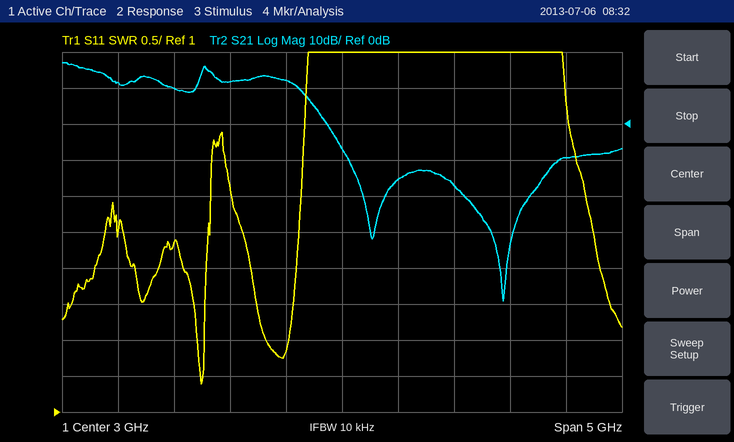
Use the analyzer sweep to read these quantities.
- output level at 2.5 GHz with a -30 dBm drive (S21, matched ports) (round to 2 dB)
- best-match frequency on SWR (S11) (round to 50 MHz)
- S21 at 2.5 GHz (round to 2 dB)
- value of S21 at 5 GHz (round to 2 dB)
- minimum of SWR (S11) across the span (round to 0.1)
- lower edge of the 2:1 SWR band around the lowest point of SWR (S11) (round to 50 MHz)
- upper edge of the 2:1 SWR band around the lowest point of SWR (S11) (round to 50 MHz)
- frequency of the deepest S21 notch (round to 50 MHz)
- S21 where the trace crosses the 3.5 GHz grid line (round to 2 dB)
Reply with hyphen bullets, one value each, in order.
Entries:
- -18 dBm
- 1.75 GHz
- 12 dB
- -10 dB
- 1.4
- 1.70 GHz
- 1.75 GHz
- 4.45 GHz
- -16 dB
